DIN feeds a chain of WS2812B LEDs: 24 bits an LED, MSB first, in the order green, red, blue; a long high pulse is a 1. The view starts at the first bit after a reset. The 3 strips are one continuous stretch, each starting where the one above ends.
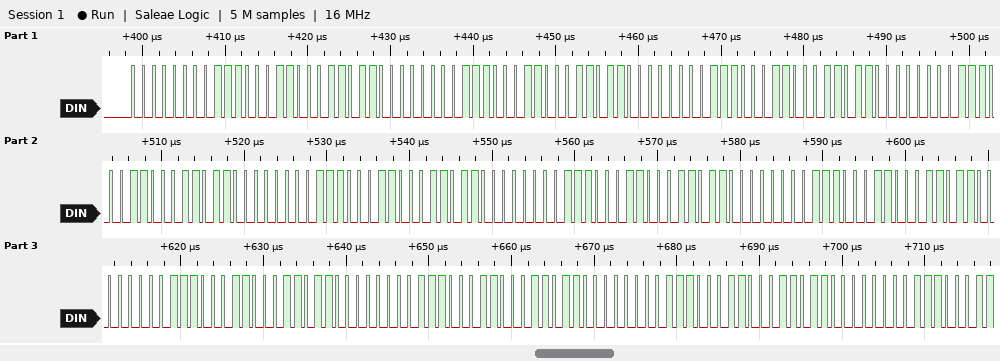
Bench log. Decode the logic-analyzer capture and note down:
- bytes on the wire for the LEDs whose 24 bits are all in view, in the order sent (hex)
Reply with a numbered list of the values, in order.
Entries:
1. 00 E3 1B 00 E3 1B 00 E3 1B 00 E3 1B 00 E3 1B 00 E3 1B 00 E3 1B 00 E3 1B 00 E3 1B 00 E3 1B
